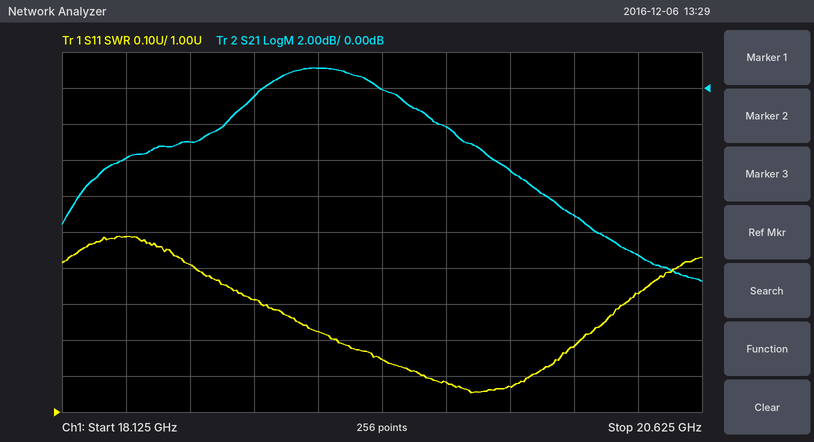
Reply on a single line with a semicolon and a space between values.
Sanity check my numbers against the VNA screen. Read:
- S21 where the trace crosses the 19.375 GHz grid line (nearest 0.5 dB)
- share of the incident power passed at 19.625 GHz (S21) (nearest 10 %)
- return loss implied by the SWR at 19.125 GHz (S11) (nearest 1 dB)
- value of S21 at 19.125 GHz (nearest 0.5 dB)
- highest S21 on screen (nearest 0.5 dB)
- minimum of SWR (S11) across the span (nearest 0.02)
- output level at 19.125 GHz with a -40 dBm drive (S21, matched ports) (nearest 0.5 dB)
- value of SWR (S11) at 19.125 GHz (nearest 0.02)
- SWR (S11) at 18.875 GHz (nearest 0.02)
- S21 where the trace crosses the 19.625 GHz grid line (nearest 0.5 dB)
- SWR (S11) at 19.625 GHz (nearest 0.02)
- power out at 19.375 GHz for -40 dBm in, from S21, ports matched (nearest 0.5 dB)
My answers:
0.0 dB; 60 %; 20 dB; 1.0 dB; 1.0 dB; 1.06; -39.0 dBm; 1.22; 1.32; -2.0 dB; 1.08; -40.0 dBm
